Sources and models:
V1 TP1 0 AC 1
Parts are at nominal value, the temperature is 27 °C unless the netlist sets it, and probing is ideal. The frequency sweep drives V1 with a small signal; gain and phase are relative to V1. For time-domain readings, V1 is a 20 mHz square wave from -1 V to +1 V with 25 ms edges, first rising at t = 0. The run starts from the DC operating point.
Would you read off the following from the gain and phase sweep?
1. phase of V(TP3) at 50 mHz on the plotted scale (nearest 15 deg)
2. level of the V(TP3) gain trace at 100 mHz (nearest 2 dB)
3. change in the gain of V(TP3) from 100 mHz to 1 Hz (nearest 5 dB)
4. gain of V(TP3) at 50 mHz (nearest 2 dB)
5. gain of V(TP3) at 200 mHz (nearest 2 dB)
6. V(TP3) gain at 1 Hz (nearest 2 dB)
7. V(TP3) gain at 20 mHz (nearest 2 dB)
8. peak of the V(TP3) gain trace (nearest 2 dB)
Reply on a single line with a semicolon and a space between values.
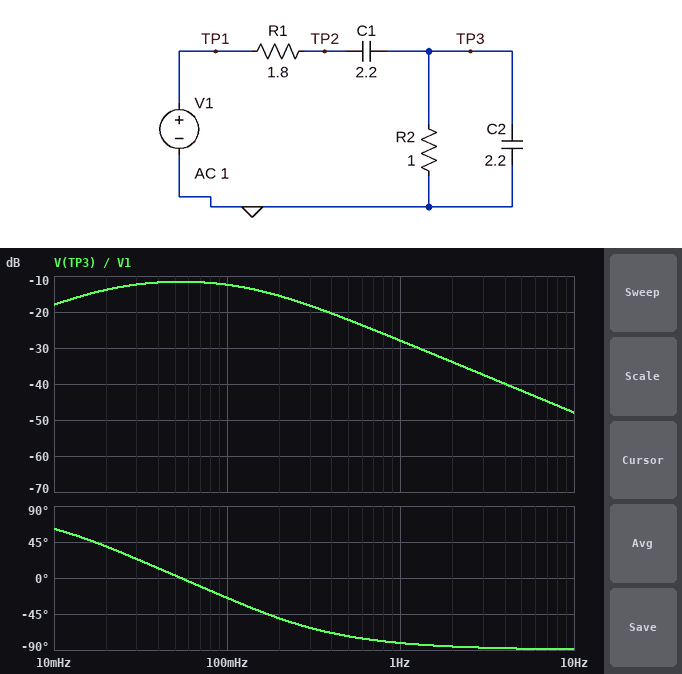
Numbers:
0 deg; -12 dB; -15 dB; -12 dB; -16 dB; -28 dB; -14 dB; -12 dB
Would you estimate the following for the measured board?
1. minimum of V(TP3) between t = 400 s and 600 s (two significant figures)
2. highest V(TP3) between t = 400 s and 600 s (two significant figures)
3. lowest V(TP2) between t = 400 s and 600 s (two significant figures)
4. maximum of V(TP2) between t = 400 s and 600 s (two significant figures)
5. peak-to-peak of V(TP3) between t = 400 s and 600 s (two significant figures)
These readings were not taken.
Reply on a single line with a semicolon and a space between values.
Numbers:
-410 mV; 410 mV; -970 mV; 970 mV; 830 mV
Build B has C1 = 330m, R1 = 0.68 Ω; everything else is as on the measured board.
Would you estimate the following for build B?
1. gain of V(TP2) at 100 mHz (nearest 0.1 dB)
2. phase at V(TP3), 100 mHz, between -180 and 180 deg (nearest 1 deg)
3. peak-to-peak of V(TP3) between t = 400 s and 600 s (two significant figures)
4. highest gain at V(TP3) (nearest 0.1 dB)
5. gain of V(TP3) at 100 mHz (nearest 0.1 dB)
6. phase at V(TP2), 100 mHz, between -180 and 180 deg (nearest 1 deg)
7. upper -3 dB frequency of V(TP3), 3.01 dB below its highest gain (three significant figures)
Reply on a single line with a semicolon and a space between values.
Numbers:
-0.1 dB; 25 deg; 420 mV; -18.4 dB; -19.3 dB; -7 deg; 942 mHz
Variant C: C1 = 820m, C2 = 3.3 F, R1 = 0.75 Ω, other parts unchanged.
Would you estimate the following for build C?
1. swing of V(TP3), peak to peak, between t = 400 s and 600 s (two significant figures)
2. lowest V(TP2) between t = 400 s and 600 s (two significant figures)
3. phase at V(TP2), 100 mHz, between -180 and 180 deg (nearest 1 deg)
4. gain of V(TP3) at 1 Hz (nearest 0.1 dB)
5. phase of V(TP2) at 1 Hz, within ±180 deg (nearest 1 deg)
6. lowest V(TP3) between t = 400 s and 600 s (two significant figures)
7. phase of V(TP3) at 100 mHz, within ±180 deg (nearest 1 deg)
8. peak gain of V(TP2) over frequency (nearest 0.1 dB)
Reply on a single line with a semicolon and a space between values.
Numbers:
580 mV; -1.0 V; -17 deg; -24.3 dB; -72 deg; -290 mV; 4 deg; 0 dB
